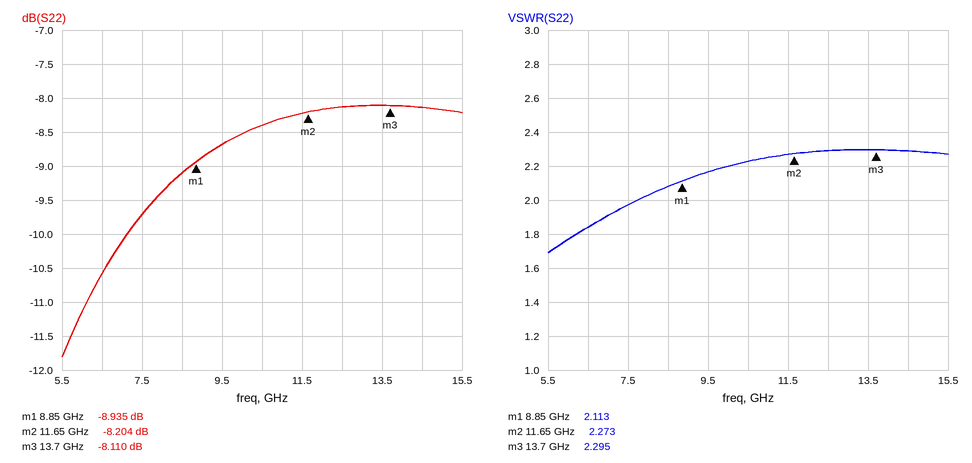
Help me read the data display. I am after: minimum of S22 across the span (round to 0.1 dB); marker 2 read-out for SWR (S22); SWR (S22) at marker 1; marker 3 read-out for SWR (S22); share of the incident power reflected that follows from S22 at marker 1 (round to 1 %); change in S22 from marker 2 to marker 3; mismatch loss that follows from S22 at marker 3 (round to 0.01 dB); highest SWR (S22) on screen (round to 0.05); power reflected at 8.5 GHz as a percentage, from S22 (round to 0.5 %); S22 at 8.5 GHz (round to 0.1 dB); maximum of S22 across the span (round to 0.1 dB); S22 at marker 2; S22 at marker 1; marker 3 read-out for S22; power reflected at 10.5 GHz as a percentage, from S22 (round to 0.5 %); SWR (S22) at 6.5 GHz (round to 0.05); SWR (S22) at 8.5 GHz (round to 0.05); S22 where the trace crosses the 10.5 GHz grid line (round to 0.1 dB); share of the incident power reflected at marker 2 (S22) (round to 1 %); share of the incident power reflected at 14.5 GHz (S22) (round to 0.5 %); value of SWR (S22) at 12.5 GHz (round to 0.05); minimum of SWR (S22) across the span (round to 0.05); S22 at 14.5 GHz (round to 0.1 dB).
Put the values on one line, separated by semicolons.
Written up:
-11.8 dB; 2.273; 2.113; 2.295; 13 %; 0.094 dB; 0.73 dB; 2.30; 12.5 %; -9.1 dB; -8.1 dB; -8.204 dB; -8.935 dB; -8.110 dB; 14.5 %; 1.85; 2.10; -8.4 dB; 15 %; 15.5 %; 2.30; 1.70; -8.1 dB
